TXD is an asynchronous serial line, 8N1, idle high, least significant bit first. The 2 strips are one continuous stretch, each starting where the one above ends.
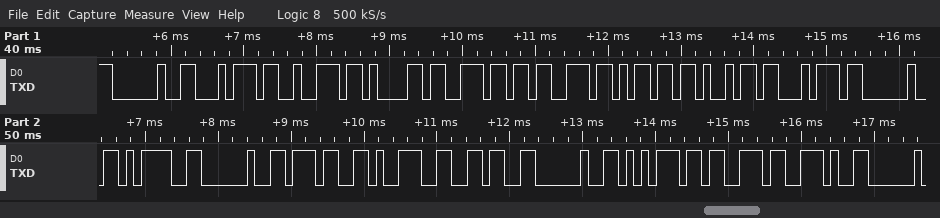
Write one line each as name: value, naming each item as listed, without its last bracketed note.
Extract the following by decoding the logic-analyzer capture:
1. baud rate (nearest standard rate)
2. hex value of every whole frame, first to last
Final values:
baud rate: 9600 baud
hex value of every whole frame, first to last: 20 74 72 61 6E 73 6D 69 74 20 3D 20 37 39 36 20 75 73 2E
